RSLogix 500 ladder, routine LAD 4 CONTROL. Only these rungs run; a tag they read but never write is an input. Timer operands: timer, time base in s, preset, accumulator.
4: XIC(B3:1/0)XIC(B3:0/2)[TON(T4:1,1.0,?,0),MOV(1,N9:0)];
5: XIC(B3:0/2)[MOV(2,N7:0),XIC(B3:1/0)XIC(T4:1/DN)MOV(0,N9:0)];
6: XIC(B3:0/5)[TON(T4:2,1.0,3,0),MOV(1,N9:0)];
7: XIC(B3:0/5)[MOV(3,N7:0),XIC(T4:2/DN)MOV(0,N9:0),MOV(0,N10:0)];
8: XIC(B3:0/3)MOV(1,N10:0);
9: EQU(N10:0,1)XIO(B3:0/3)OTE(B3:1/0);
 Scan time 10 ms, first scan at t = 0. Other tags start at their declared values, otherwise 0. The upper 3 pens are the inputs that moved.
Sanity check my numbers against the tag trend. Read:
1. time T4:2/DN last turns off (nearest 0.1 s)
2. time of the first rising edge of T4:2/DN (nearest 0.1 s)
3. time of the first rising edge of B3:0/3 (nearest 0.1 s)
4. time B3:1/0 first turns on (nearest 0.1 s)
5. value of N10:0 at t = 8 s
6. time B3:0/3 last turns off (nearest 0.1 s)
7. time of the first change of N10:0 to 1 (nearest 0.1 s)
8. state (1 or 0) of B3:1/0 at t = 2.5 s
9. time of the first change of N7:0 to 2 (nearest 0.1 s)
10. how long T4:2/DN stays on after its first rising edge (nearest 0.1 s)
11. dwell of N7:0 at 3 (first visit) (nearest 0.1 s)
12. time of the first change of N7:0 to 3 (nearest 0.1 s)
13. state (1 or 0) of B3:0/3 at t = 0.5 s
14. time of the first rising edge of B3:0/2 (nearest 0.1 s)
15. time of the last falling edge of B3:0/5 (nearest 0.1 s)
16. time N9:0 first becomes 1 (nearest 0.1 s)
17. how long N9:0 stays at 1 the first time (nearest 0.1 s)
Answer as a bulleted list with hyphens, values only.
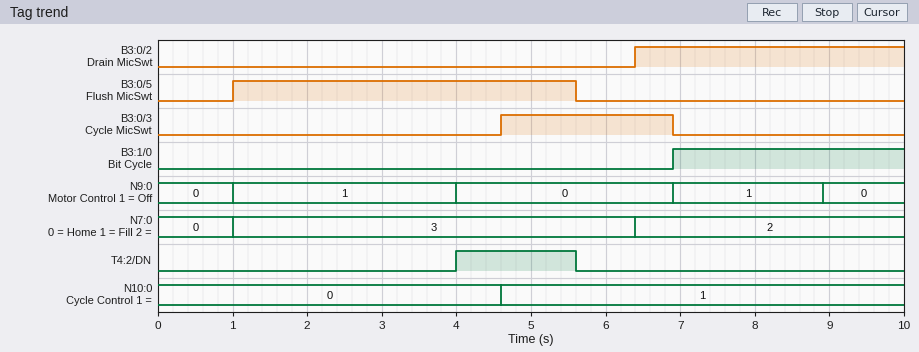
- 5.6 s
- 4.0 s
- 4.6 s
- 6.9 s
- 1
- 6.9 s
- 4.6 s
- 0
- 6.4 s
- 1.6 s
- 5.4 s
- 1.0 s
- 0
- 6.4 s
- 5.6 s
- 1.0 s
- 3.0 s
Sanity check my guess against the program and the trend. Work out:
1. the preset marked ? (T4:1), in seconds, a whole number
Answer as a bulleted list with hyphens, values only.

- 2 s
